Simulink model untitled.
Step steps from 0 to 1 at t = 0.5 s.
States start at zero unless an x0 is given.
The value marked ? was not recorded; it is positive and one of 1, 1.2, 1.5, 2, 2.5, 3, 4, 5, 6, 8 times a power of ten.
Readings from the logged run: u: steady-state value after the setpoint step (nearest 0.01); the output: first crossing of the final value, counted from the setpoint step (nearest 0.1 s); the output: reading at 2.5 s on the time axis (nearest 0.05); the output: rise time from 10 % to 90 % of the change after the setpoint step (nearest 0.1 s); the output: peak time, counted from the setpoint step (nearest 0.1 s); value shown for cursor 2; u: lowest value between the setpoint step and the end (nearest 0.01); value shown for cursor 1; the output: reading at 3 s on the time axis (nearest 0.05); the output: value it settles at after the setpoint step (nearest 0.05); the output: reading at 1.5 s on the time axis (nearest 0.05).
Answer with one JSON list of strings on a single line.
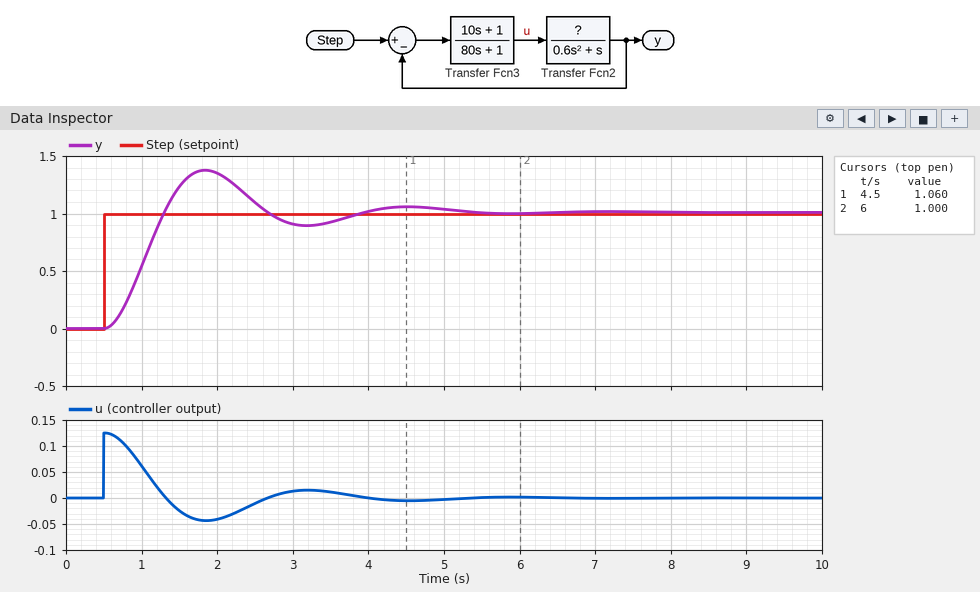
["0.00", "0.8 s", "1.10", "0.5 s", "1.3 s", "1.000", "-0.04", "1.060", "0.90", "1.00", "1.25"]
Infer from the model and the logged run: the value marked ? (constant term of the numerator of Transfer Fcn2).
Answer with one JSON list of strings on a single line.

["30"]
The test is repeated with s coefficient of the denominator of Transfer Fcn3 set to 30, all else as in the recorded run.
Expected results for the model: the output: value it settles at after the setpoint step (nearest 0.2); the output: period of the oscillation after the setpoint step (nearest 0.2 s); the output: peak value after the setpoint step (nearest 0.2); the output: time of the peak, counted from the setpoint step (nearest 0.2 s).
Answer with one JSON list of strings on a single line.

["1.0", "1.6 s", "1.6", "0.8 s"]
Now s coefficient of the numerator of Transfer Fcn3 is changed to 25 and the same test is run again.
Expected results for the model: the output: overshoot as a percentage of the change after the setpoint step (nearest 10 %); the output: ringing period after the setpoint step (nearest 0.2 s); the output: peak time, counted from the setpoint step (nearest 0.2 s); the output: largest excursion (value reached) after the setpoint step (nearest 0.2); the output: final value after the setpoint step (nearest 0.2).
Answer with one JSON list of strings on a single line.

["50 %", "1.6 s", "0.8 s", "1.6", "1.0"]
